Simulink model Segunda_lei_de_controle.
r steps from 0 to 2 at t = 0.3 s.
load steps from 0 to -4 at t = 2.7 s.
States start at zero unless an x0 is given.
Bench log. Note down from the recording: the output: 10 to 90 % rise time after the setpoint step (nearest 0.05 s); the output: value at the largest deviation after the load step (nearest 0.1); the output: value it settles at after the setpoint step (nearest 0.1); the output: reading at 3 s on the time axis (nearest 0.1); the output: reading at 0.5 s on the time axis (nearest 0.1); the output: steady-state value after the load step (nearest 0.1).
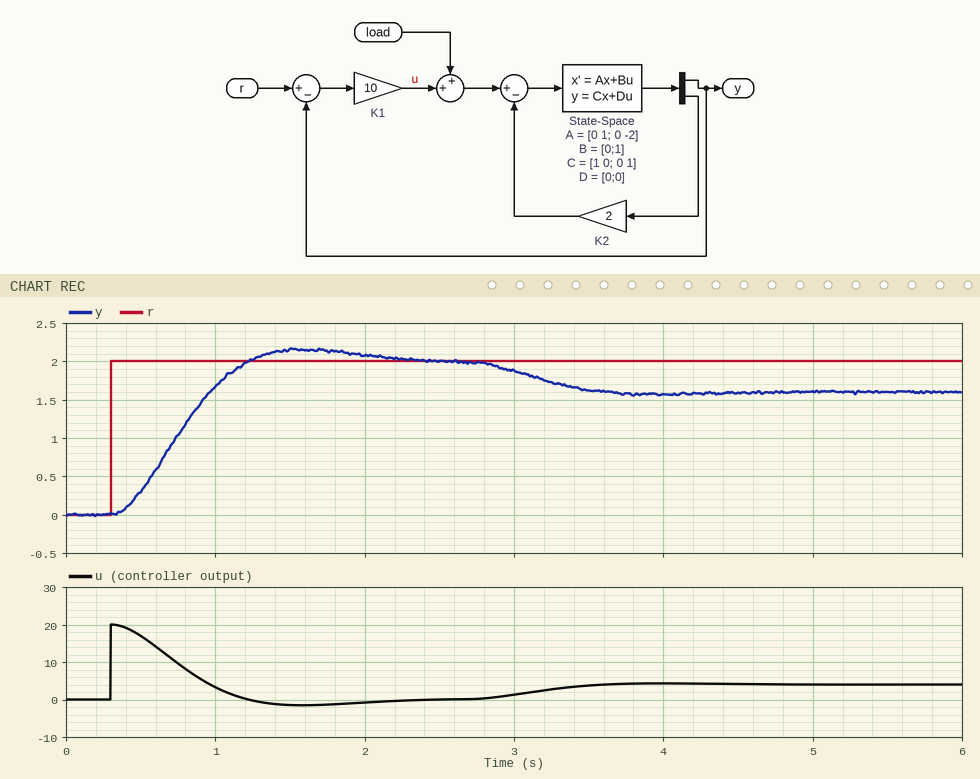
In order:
0.60 s
1.6
2.0
1.9
0.3
1.6
